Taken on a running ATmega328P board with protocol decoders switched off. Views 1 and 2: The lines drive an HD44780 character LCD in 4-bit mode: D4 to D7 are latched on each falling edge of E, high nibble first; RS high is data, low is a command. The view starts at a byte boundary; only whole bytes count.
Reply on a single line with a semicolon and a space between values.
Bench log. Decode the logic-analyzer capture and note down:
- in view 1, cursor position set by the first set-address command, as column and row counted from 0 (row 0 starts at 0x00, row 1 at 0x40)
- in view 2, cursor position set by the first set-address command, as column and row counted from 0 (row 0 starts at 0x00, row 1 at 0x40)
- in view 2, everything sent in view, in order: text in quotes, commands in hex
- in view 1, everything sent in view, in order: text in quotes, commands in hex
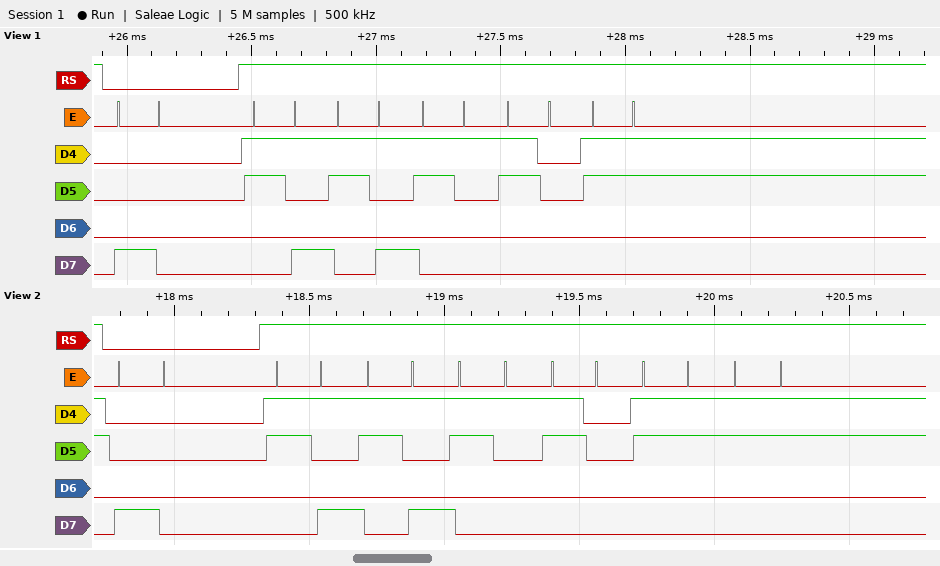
column 0, row 0; column 0, row 0; 0x80 "991033"; 0x80 "99103"
